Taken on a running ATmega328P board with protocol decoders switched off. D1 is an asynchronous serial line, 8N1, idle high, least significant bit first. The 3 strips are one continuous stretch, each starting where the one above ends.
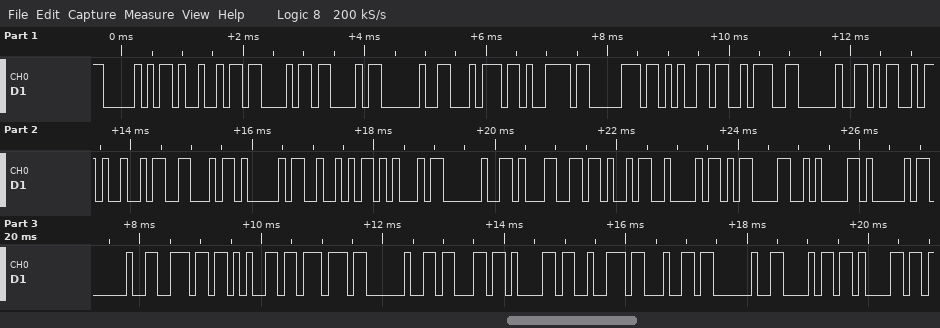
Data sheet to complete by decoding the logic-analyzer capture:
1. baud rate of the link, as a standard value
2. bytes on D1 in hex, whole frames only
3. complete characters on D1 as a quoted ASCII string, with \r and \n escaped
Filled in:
9600 baud
50 49 43 43 20 74 79 70 65 3A 20 4D 49 46 41 52 45 20 31 4B 42 0D 0A 41 20 6E 65 77 20 63 61 72 64 20 68 61
"PICC type: MIFARE 1KB\r\nA new card ha"
